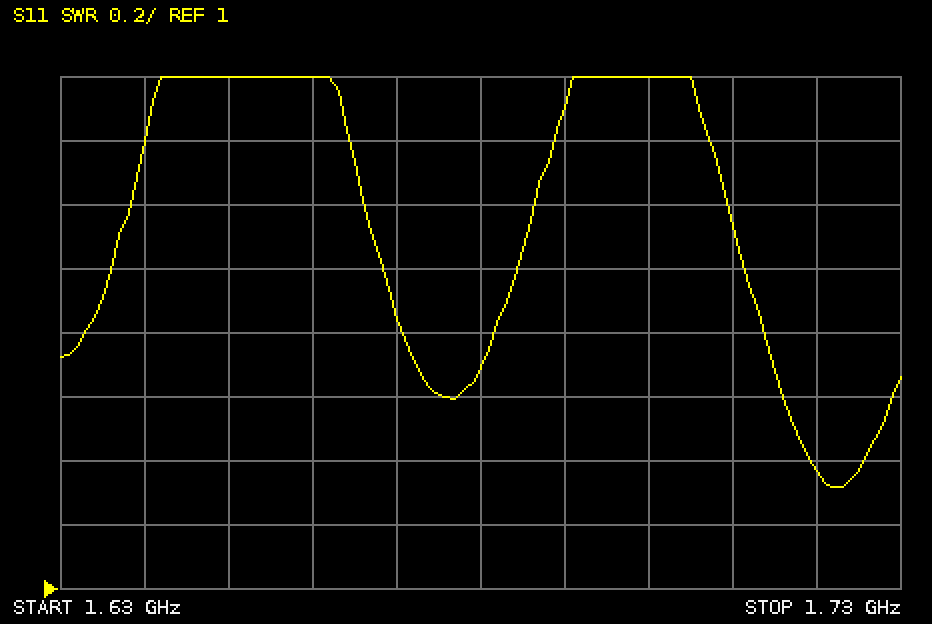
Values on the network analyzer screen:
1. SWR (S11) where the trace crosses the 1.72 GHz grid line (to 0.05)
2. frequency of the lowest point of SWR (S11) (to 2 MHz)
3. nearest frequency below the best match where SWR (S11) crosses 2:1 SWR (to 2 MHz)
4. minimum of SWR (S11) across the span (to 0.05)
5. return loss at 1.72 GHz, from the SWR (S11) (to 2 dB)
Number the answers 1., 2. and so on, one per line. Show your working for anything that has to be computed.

1. 1.35
2. 1.722 GHz
3. 1.712 GHz
4. 1.30
5. −20 log10((1.35 − 1)/(1.35 + 1)) ≈ 16 dB
